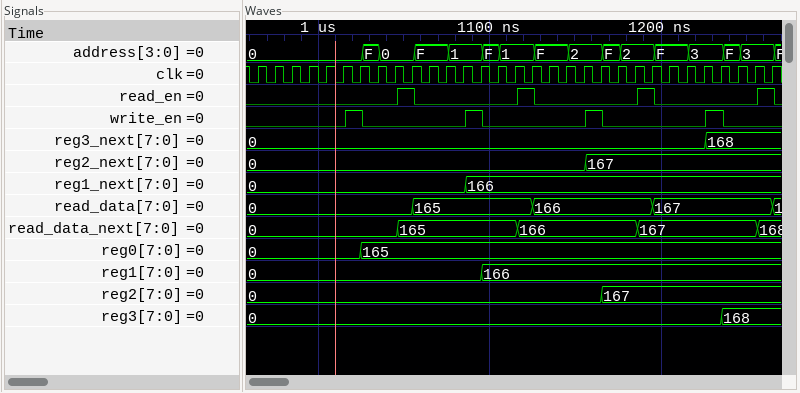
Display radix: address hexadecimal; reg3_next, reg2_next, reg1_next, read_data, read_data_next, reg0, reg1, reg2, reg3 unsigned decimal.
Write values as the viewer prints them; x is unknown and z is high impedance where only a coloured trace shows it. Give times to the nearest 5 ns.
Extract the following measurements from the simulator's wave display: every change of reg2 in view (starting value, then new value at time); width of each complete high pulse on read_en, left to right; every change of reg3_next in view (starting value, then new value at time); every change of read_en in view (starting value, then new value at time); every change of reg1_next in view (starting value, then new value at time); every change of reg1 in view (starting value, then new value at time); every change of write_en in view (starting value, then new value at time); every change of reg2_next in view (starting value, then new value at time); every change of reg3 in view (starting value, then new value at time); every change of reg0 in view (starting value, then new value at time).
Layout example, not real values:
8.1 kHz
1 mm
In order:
0, 167 at 1165 ns
10 ns, 10 ns, 10 ns, 10 ns
0, 168 at 1225 ns
0, 1 at 1045 ns, 0 at 1055 ns, 1 at 1115 ns, 0 at 1125 ns, 1 at 1185 ns, 0 at 1195 ns, 1 at 1255 ns, 0 at 1265 ns
0, 166 at 1085 ns
0, 166 at 1095 ns
0, 1 at 1015 ns, 0 at 1025 ns, 1 at 1085 ns, 0 at 1095 ns, 1 at 1155 ns, 0 at 1165 ns, 1 at 1225 ns, 0 at 1235 ns
0, 167 at 1155 ns
0, 168 at 1235 ns
0, 165 at 1025 ns
